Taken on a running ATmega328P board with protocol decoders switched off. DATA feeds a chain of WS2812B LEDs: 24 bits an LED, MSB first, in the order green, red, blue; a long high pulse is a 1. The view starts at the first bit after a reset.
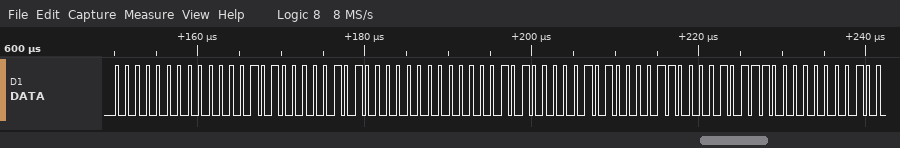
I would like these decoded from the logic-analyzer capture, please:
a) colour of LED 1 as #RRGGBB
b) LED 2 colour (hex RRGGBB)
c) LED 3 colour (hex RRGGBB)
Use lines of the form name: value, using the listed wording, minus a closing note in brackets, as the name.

colour of LED 1 as #RRGGBB: #050005
LED 2 colour: #050005
LED 3 colour: #2E0C01
